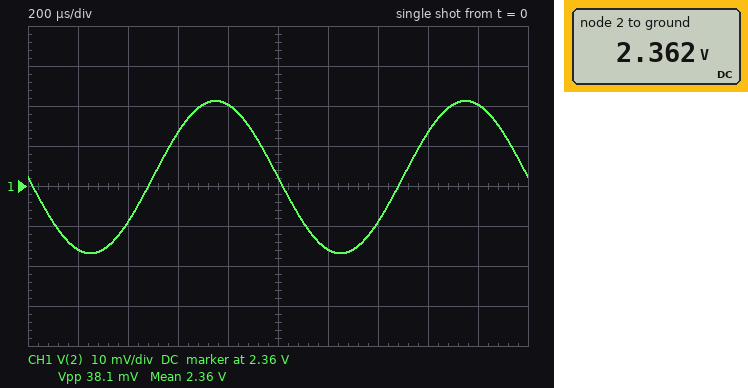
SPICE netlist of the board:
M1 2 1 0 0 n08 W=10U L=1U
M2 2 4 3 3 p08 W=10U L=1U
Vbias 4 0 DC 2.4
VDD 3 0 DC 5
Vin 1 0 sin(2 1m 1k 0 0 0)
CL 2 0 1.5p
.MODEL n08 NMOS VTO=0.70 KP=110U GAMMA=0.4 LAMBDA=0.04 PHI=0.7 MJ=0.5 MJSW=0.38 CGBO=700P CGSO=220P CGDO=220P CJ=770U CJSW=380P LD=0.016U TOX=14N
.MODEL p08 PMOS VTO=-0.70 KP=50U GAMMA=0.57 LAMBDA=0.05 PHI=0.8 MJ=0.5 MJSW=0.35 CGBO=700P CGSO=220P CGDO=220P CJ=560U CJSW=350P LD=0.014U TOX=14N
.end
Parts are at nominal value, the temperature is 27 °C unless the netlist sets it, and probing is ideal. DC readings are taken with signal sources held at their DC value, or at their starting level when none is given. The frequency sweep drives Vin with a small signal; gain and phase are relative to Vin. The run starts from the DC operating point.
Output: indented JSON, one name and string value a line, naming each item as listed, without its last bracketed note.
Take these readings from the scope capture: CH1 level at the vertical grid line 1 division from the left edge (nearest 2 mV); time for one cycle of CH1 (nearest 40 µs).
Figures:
{
  "CH1 level at the vertical grid line 1 division from the left edge": "2.344 V",
  "time for one cycle of CH1": "1.00 ms"
}
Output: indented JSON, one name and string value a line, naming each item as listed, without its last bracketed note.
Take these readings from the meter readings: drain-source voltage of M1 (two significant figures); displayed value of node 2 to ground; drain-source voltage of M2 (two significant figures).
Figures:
{
  "drain-source voltage of M1": "2.4 V",
  "displayed value of node 2 to ground": "2.362 V",
  "drain-source voltage of M2": "-2.6 V"
}
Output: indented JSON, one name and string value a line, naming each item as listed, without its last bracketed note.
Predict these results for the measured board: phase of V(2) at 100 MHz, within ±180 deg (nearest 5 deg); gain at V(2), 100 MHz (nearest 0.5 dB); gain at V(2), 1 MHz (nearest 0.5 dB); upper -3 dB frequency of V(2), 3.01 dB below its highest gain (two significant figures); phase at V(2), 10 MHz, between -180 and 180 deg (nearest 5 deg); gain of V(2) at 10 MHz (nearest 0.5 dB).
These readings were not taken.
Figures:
{
  "phase of V(2) at 100 MHz, within ±180 deg": "95 deg",
  "gain at V(2), 100 MHz": "4.5 dB",
  "gain at V(2), 1 MHz": "25.5 dB",
  "upper -3 dB frequency of V(2), 3.01 dB below its highest gain": "9.0 MHz",
  "phase at V(2), 10 MHz, between -180 and 180 deg": "130 deg",
  "gain of V(2) at 10 MHz": "22.0 dB"
}
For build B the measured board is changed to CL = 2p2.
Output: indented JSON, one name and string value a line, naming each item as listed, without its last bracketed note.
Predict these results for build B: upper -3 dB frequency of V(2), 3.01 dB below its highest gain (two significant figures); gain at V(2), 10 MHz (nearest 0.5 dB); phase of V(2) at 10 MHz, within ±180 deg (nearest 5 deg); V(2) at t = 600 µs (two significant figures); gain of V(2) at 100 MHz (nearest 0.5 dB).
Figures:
{
  "upper -3 dB frequency of V(2), 3.01 dB below its highest gain": "6.1 MHz",
  "gain at V(2), 10 MHz": "20.0 dB",
  "phase of V(2) at 10 MHz, within ±180 deg": "120 deg",
  "V(2) at t = 600 µs": "2.4 V",
  "gain of V(2) at 100 MHz": "1.5 dB"
}
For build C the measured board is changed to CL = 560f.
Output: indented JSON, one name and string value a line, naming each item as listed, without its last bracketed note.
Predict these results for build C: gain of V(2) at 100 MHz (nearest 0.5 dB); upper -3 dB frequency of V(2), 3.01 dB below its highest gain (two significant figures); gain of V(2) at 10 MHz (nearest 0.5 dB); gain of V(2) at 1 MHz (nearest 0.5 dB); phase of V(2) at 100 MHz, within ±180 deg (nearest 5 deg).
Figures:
{
  "gain of V(2) at 100 MHz": "13.0 dB",
  "upper -3 dB frequency of V(2), 3.01 dB below its highest gain": "24 MHz",
  "gain of V(2) at 10 MHz": "25.0 dB",
  "gain of V(2) at 1 MHz": "25.5 dB",
  "phase of V(2) at 100 MHz, within ±180 deg": "105 deg"
}
